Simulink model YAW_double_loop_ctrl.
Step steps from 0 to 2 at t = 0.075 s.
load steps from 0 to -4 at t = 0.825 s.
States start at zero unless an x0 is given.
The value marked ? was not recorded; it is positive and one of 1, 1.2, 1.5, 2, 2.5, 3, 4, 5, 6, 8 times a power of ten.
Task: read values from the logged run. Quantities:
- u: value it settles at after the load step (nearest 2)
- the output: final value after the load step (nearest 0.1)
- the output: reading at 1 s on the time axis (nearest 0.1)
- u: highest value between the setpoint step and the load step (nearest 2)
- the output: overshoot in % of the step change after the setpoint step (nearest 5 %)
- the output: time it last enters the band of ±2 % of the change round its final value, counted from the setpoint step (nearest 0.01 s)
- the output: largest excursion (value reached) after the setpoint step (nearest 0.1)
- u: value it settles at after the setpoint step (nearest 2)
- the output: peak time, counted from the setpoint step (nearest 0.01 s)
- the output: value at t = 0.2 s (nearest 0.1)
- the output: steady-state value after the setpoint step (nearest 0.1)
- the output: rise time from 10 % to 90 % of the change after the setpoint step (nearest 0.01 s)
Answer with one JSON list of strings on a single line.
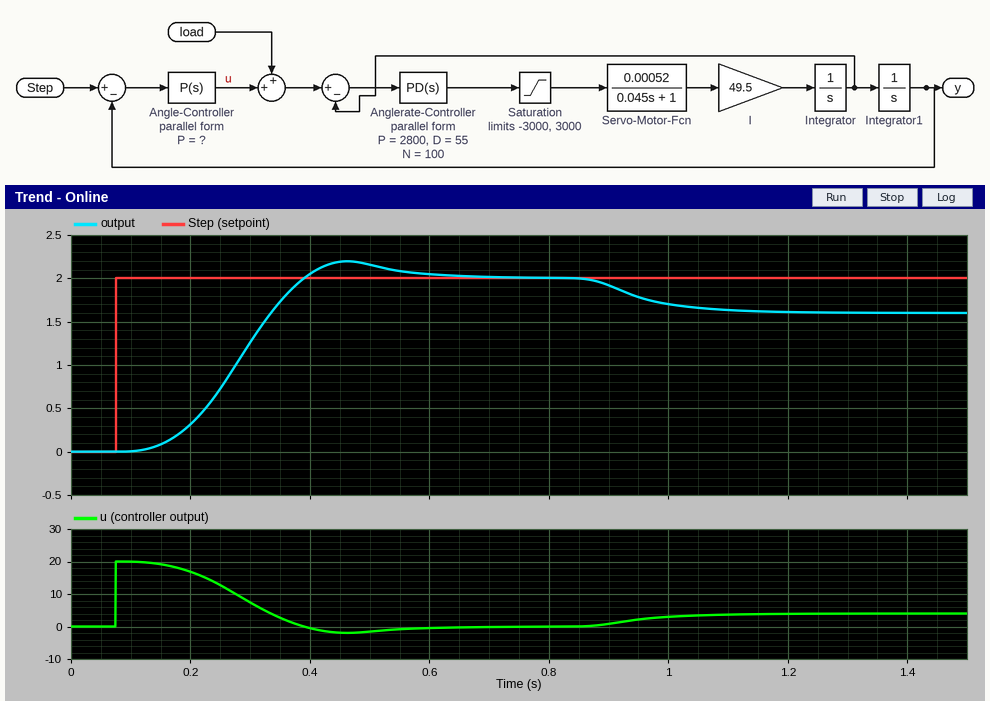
["4", "1.6", "1.7", "20", "10 %", "0.54 s", "2.2", "0", "0.39 s", "0.3", "2.0", "0.18 s"]
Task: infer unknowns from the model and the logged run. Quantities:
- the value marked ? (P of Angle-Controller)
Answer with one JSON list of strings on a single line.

["10"]
